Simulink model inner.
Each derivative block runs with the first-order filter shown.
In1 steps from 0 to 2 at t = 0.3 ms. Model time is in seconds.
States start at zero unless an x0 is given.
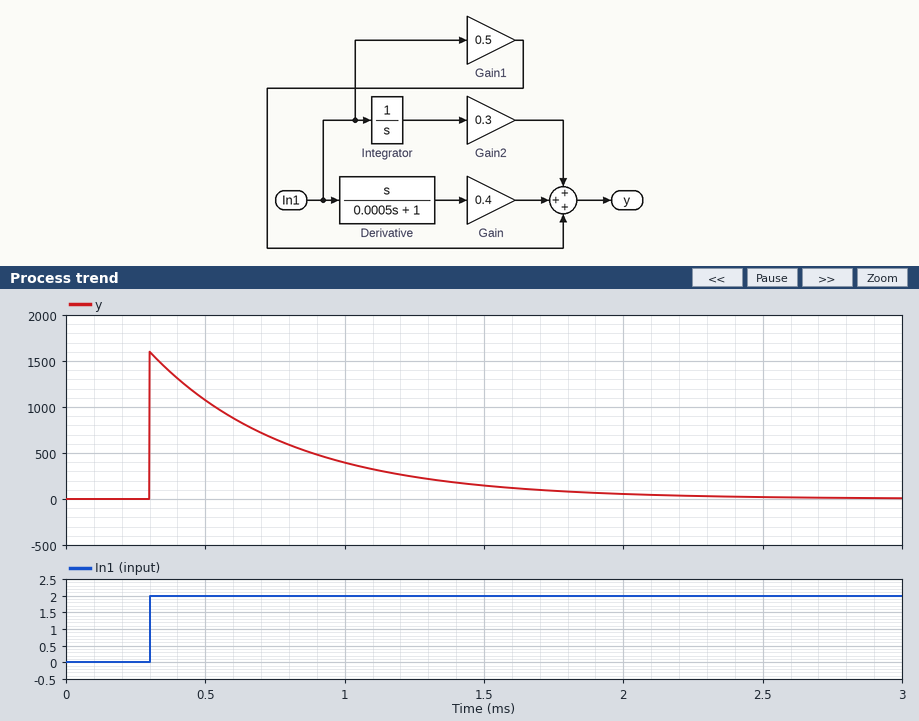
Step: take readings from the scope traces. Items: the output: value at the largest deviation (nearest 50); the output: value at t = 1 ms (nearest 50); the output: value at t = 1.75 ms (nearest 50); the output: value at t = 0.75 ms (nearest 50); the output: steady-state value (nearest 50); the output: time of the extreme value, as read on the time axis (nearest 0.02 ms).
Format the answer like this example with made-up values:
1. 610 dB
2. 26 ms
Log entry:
1. 1600
2. 400
3. 100
4. 650
5. 0
6. 0.30 ms
